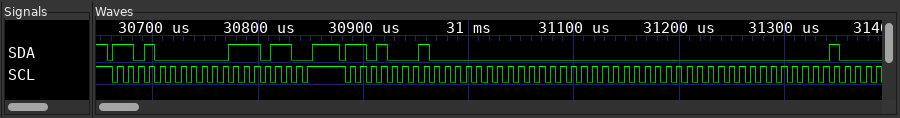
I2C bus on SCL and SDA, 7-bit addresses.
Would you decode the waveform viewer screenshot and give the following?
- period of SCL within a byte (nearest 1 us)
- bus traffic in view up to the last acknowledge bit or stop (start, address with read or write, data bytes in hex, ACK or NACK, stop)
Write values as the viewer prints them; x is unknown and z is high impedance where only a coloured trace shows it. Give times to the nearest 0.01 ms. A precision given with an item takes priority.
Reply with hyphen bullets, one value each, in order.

- 10 us
- start, address 68 write ACK, 3B ACK, stop, start, address 68 read ACK, 00 ACK, 00 ACK, 00 ACK, 00 ACK
